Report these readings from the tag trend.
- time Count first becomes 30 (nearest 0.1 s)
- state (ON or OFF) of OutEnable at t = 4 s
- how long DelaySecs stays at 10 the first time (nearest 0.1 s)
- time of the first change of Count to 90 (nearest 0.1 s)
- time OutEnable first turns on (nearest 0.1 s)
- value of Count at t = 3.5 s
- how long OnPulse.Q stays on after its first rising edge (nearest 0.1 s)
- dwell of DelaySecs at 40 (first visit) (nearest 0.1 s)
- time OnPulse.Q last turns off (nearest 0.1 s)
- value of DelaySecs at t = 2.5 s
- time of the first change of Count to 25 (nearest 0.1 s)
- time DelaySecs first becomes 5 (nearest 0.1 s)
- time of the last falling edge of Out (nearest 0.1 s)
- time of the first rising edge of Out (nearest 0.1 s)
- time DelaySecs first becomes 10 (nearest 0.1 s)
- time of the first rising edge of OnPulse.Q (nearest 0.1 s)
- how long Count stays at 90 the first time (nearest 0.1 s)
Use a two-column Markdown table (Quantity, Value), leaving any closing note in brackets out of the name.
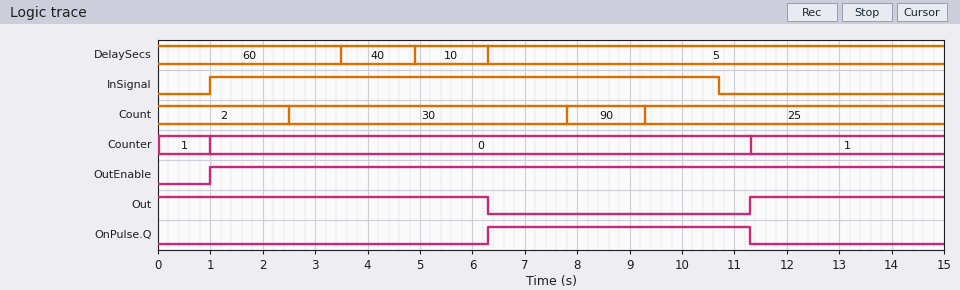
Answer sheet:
| Quantity | Value |
|---|---|
| time Count first becomes 30 | 2.5 s |
| state (ON or OFF) of OutEnable at t = 4 s | ON |
| how long DelaySecs stays at 10 the first time | 1.4 s |
| time of the first change of Count to 90 | 7.8 s |
| time OutEnable first turns on | 1.0 s |
| value of Count at t = 3.5 s | 30 |
| how long OnPulse.Q stays on after its first rising edge | 5.0 s |
| dwell of DelaySecs at 40 (first visit) | 1.4 s |
| time OnPulse.Q last turns off | 11.3 s |
| value of DelaySecs at t = 2.5 s | 60 |
| time of the first change of Count to 25 | 9.3 s |
| time DelaySecs first becomes 5 | 6.3 s |
| time of the last falling edge of Out | 6.3 s |
| time of the first rising edge of Out | 11.3 s |
| time DelaySecs first becomes 10 | 4.9 s |
| time of the first rising edge of OnPulse.Q | 6.3 s |
| how long Count stays at 90 the first time | 1.5 s |
